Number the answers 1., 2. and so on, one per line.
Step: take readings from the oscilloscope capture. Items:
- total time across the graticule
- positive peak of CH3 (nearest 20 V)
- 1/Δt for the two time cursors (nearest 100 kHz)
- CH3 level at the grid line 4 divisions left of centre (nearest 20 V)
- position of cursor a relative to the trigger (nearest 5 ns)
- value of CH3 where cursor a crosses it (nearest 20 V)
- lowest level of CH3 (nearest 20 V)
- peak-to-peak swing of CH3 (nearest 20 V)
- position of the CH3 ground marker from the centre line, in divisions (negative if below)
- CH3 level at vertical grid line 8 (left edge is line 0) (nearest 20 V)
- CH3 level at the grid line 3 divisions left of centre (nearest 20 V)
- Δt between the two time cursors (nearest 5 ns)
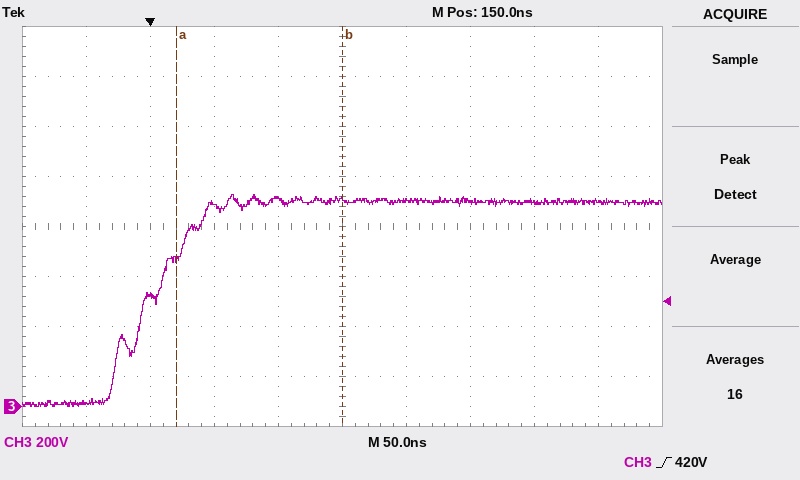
1. 500 ns
2. 840 V
3. 7.7 MHz
4. 20 V
5. +20 ns
6. 580 V
7. 0 V
8. 840 V
9. -3.6 div
10. 820 V
11. 440 V
12. 130 ns
